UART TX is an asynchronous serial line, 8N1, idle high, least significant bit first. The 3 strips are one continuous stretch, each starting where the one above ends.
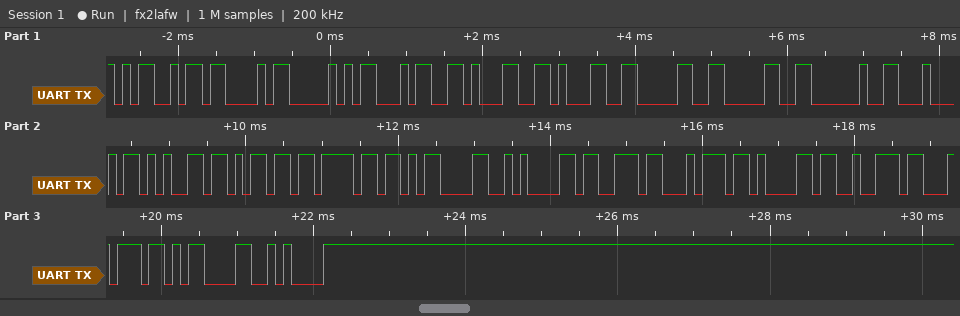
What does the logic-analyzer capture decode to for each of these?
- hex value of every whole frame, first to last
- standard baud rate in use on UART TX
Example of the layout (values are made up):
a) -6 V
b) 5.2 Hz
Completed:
a) 4D 43 50 34 31 31 30 30 20 44 65 6D 6F 0D 0A 73 74 61 72 74 0D 0A
b) 9600 baud
